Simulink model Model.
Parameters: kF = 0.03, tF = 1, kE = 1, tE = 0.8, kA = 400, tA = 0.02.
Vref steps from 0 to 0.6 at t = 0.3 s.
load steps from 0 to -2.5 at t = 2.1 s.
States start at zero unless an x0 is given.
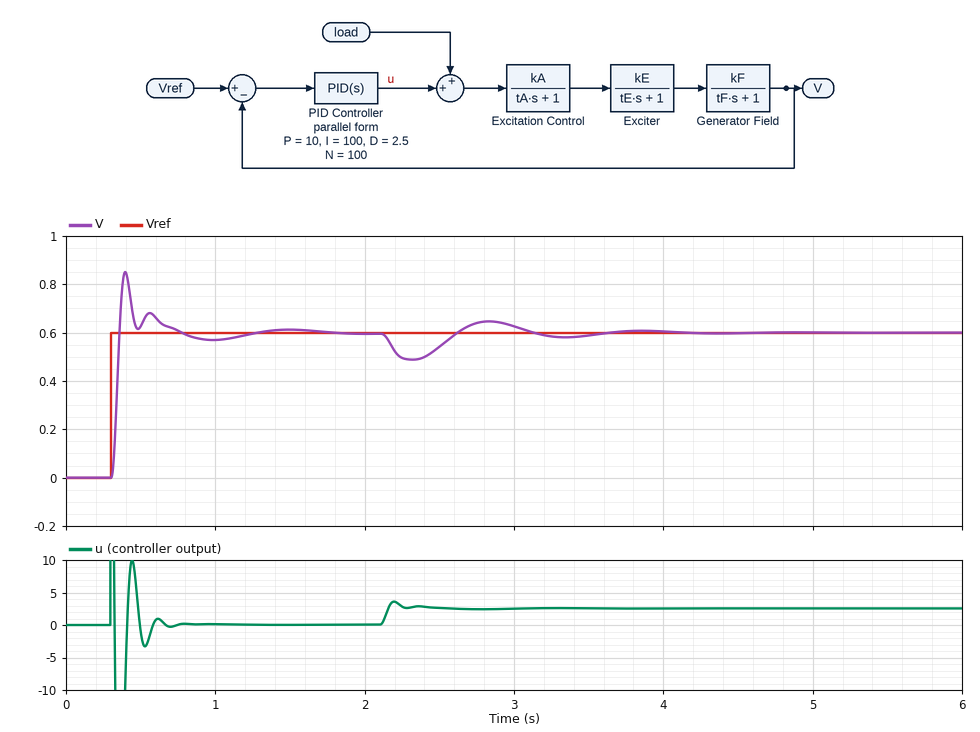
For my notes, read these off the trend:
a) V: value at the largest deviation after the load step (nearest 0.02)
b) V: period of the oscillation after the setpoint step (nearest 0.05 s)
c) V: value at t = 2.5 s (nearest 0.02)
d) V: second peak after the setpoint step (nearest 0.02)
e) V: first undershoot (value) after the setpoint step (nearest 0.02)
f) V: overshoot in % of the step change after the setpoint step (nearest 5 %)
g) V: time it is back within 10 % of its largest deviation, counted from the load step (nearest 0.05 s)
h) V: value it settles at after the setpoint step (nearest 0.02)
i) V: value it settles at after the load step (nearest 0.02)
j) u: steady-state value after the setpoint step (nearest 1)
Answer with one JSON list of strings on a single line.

["0.48", "0.15 s", "0.54", "0.68", "0.62", "40 %", "1.40 s", "0.60", "0.60", "0"]
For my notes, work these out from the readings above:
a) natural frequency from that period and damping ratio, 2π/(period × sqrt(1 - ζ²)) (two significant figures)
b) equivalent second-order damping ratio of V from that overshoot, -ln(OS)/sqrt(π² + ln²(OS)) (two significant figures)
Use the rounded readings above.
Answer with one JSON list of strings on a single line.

["44 rad/s", "0.28"]
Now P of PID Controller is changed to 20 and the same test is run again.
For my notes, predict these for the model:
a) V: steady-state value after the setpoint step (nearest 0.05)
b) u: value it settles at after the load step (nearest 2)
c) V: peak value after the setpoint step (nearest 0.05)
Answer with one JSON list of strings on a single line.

["0.60", "2", "0.95"]
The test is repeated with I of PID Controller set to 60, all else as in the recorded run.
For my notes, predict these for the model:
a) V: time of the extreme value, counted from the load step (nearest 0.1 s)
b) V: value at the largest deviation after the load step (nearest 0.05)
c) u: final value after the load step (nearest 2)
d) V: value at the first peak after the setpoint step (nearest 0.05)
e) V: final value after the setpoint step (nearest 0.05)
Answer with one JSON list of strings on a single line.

["0.3 s", "0.45", "2", "0.85", "0.60"]
